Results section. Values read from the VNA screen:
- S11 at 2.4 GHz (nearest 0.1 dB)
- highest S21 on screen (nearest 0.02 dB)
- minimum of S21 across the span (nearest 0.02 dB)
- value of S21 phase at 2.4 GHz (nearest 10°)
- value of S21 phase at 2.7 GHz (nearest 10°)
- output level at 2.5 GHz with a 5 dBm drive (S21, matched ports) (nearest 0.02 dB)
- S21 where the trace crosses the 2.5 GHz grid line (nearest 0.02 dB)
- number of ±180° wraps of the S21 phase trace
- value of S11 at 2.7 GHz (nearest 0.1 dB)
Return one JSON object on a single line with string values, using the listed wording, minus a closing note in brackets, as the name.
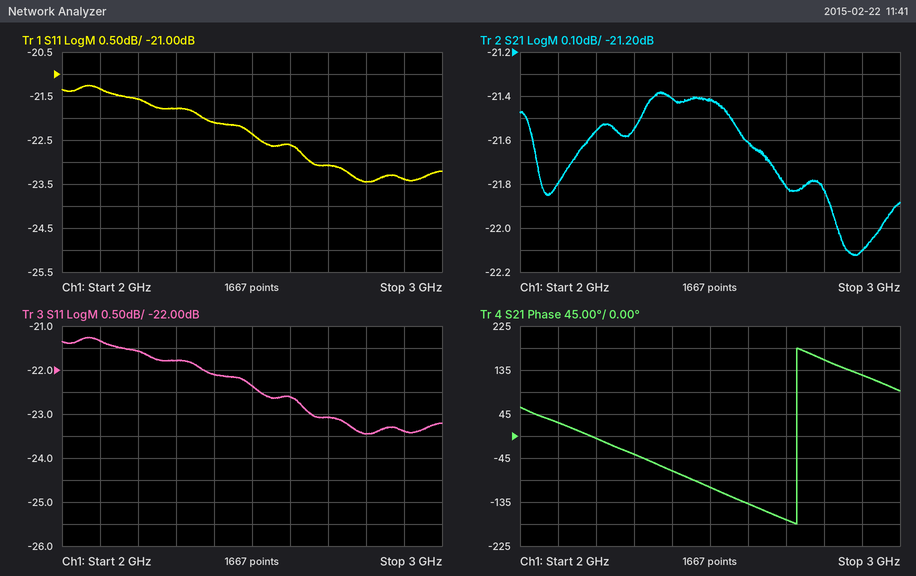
{"S11 at 2.4 GHz": "-22.1 dB", "highest S21 on screen": "-21.38 dB", "minimum of S21 across the span": "-22.12 dB", "value of S21 phase at 2.4 GHz": "-70°", "value of S21 phase at 2.7 GHz": "-170°", "output level at 2.5 GHz with a 5 dBm drive (S21, matched ports)": "-16.42 dBm", "S21 where the trace crosses the 2.5 GHz grid line": "-21.42 dB", "number of ±180° wraps of the S21 phase trace": "1", "value of S11 at 2.7 GHz": "-23.1 dB"}
